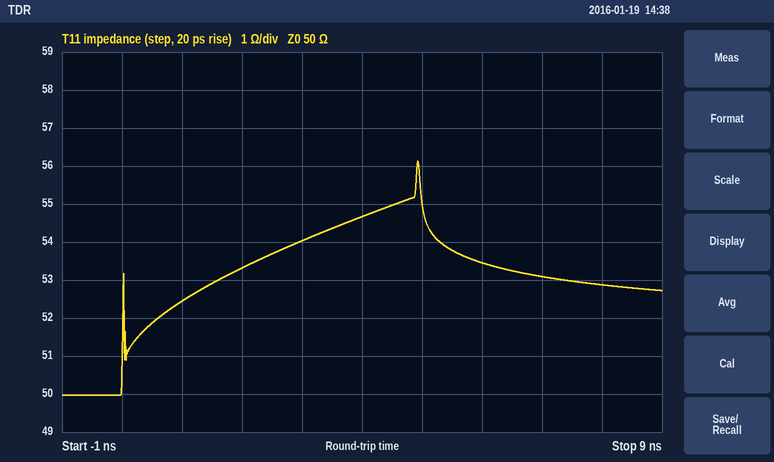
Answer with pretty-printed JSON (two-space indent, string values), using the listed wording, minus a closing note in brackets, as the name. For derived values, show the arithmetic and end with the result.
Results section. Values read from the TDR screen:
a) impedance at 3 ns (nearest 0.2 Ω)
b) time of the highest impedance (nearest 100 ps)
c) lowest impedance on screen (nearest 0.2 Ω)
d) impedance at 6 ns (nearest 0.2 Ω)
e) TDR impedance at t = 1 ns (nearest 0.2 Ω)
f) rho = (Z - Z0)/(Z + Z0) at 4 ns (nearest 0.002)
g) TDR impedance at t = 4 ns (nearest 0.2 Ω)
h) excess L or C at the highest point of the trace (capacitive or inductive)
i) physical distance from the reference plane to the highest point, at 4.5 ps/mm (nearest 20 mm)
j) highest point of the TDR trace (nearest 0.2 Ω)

{
  "impedance at 3 ns": "54.0 Ω",
  "time of the highest impedance": "4.9 ns",
  "lowest impedance on screen": "50.0 Ω",
  "impedance at 6 ns": "53.4 Ω",
  "TDR impedance at t = 1 ns": "52.4 Ω",
  "rho = (Z - Z0)/(Z + Z0) at 4 ns": "(54.6 − 50)/(54.6 + 50) ≈ +0.044",
  "TDR impedance at t = 4 ns": "54.6 Ω",
  "excess L or C at the highest point of the trace": "inductive",
  "physical distance from the reference plane to the highest point, at 4.5 ps/mm": "4.9 ns / 2 / 4.5 ps/mm ≈ 544 mm, so 540 mm to the nearest 20 mm",
  "highest point of the TDR trace": "56.2 Ω"
}
